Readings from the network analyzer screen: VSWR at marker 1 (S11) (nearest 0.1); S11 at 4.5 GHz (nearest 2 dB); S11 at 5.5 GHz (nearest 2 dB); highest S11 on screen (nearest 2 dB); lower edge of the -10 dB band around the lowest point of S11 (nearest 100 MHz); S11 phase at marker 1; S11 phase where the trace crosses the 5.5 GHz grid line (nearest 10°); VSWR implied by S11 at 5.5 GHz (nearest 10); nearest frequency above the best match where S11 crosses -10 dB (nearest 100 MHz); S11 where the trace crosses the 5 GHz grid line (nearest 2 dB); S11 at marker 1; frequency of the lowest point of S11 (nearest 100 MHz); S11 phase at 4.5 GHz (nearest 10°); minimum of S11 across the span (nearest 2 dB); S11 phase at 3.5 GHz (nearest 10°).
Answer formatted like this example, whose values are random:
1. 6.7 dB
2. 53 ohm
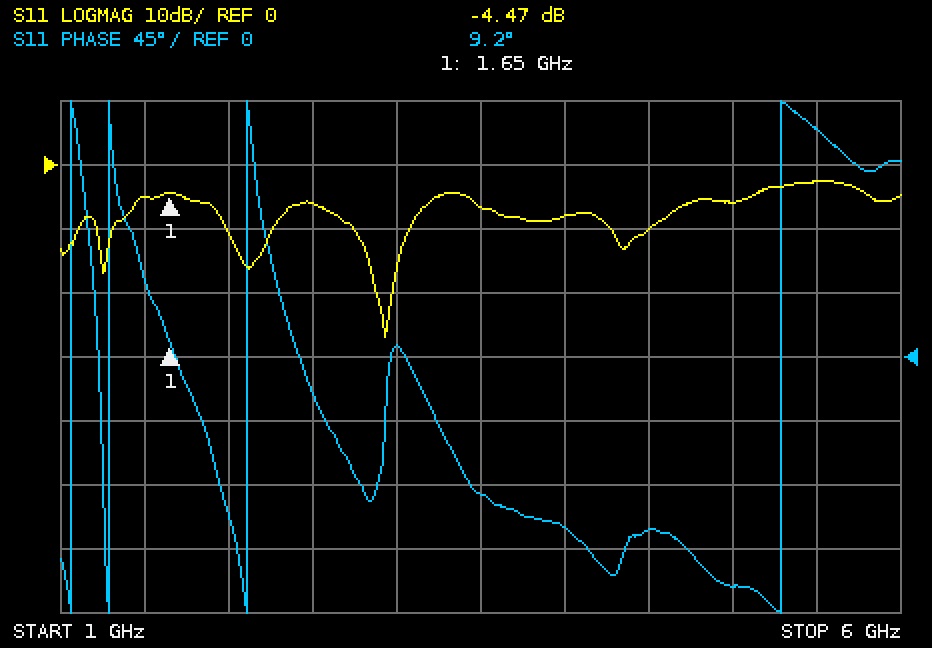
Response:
1. 4.0
2. -10 dB
3. -2 dB
4. -2 dB
5. 2.7 GHz
6. 9.2°
7. 160°
8. 10
9. 3.1 GHz
10. -6 dB
11. -4.47 dB
12. 2.9 GHz
13. -120°
14. -26 dB
15. -100°
